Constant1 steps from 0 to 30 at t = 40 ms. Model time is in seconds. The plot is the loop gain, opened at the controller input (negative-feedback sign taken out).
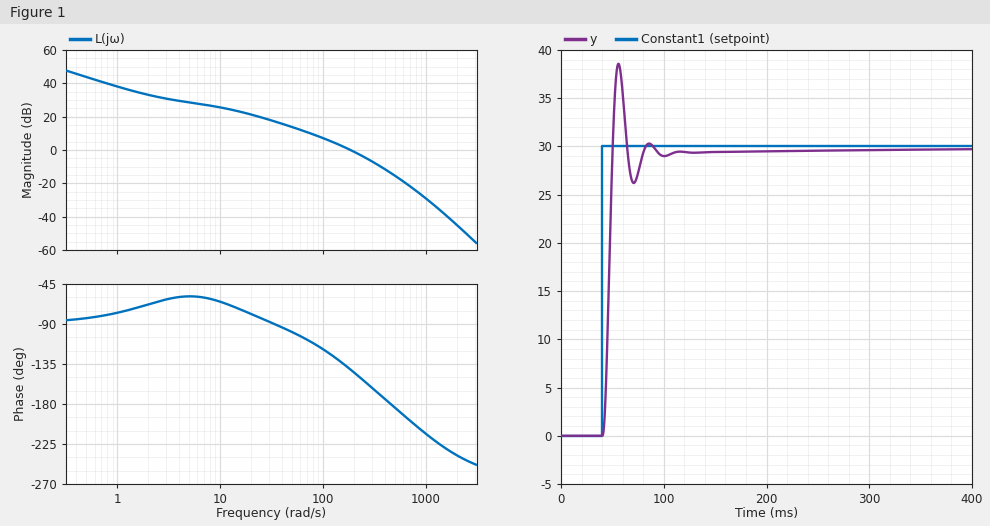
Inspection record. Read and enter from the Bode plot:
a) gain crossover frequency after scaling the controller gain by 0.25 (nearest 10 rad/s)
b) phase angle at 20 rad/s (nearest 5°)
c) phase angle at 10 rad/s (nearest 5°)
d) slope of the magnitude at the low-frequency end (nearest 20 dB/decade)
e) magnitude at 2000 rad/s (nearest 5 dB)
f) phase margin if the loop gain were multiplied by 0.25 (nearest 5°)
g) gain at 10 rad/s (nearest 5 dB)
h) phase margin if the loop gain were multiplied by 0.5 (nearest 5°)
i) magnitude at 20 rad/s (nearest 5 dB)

60 rad/s
-80°
-65°
-20 dB/decade
-45 dB
75°
25 dB
60°
20 dB
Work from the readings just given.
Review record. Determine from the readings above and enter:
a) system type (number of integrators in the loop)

1
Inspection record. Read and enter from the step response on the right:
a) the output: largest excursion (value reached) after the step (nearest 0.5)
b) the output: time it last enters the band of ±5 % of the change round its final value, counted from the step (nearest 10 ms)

38.5
40 ms
